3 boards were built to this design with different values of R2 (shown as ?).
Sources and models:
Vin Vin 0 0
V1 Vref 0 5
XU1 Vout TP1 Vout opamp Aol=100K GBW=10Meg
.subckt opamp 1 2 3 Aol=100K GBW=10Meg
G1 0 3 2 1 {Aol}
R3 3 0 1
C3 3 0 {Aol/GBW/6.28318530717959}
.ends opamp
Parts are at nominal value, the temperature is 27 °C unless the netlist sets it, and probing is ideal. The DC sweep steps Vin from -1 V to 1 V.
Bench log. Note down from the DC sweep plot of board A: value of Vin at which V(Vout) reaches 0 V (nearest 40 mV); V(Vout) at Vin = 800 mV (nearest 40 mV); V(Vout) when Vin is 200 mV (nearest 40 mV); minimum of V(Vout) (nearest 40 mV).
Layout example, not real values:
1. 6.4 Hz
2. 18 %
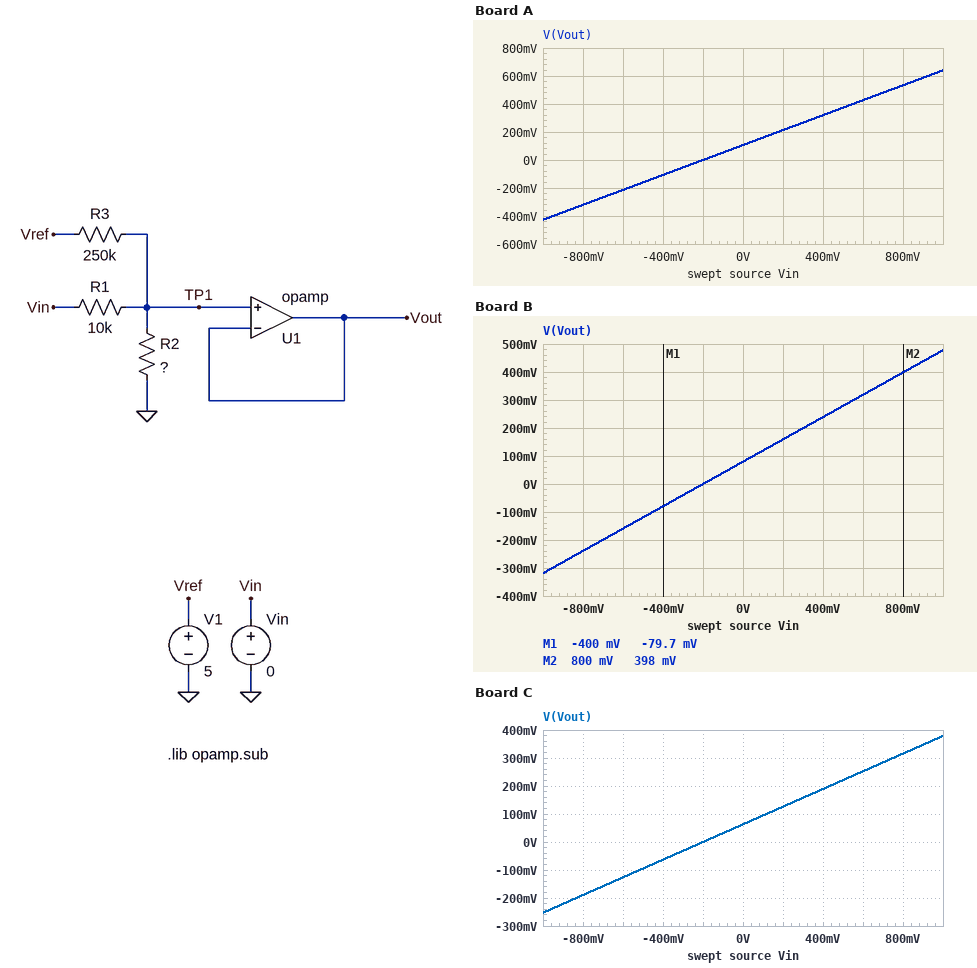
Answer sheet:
1. -200 mV
2. 520 mV
3. 200 mV
4. -440 mV
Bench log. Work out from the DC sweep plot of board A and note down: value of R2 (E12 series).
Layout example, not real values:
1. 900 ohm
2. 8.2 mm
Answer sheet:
1. 12 kΩ
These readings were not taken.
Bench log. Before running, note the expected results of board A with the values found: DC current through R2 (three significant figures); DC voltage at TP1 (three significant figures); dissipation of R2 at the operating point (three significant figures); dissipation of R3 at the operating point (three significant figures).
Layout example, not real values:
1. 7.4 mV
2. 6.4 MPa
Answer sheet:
1. 8.90 µA
2. 107 mV
3. 950 nW
4. 95.8 µW
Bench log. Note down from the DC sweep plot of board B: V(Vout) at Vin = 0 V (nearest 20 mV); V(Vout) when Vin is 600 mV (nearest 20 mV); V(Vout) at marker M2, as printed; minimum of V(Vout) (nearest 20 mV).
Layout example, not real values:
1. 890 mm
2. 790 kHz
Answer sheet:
1. 80 mV
2. 320 mV
3. 398 mV
4. -320 mV
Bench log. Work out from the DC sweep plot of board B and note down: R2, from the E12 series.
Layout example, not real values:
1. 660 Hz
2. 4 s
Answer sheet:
1. 6.8 kΩ
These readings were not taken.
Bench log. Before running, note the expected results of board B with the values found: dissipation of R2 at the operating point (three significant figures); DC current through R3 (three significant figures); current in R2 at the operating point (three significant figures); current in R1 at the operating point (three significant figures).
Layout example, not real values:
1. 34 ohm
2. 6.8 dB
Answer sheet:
1. 933 nW
2. 19.7 µA
3. 11.7 µA
4. 7.97 µA
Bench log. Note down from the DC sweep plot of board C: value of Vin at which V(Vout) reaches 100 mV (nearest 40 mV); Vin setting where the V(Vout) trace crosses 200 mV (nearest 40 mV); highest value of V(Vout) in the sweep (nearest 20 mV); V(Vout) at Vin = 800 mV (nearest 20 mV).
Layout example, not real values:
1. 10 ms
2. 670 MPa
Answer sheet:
1. 120 mV
2. 440 mV
3. 380 mV
4. 320 mV
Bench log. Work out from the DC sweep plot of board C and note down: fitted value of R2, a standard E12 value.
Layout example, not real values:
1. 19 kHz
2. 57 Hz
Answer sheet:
1. 4.7 kΩ
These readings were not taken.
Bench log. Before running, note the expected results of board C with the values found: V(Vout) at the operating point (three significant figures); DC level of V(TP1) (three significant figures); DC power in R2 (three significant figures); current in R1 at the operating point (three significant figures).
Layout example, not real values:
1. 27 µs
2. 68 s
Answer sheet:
1. 63.1 mV
2. 63.1 mV
3. 848 nW
4. 6.31 µA
